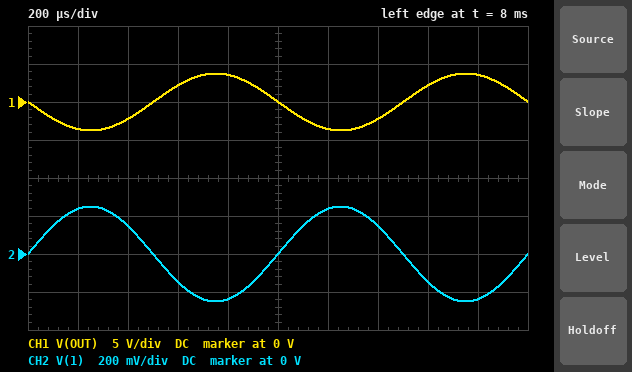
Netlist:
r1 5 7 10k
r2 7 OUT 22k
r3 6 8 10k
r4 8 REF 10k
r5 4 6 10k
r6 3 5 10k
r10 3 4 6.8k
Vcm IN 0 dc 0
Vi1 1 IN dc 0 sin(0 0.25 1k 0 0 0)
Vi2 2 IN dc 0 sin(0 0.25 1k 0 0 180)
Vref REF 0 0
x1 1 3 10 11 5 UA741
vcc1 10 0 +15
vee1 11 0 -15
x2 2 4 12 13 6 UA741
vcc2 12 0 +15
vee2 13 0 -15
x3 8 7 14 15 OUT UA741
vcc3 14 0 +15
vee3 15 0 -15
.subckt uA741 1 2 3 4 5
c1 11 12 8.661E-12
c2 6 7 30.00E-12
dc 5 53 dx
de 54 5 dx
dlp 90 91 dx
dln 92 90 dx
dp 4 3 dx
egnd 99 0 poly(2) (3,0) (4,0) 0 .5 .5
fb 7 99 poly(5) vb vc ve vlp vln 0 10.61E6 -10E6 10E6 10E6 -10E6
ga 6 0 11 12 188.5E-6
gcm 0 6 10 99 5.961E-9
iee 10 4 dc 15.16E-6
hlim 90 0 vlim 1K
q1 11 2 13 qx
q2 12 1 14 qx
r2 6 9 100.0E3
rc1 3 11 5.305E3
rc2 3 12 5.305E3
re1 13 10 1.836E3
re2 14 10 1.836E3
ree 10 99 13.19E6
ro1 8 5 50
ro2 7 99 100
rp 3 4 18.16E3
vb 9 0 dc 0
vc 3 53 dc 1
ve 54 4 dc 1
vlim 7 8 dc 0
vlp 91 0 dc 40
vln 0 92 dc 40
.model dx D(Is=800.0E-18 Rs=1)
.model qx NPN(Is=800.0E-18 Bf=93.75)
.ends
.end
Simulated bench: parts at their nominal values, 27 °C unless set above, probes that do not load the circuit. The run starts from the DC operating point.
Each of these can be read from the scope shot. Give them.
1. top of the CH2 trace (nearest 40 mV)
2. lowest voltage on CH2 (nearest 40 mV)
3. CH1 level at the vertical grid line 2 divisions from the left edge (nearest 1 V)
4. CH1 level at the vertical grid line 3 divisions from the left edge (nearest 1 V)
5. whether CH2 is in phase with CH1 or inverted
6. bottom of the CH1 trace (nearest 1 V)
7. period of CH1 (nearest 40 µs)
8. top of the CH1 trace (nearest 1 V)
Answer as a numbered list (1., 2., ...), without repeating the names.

1. 240 mV
2. -240 mV
3. -2 V
4. 2 V
5. inverted
6. -4 V
7. 1.00 ms
8. 4 V
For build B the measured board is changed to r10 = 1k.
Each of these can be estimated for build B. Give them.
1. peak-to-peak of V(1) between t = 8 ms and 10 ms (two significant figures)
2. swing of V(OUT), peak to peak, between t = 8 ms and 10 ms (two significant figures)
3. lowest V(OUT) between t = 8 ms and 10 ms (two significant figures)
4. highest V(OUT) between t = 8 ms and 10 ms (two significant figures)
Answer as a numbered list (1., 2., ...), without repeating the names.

1. 500 mV
2. 29 V
3. -15 V
4. 15 V
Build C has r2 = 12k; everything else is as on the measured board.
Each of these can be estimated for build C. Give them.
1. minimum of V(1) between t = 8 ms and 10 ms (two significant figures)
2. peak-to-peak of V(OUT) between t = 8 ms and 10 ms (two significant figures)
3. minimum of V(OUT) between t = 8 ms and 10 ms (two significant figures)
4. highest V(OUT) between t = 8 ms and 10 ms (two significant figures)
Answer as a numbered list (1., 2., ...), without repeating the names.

1. -250 mV
2. 4.5 V
3. -2.3 V
4. 2.3 V
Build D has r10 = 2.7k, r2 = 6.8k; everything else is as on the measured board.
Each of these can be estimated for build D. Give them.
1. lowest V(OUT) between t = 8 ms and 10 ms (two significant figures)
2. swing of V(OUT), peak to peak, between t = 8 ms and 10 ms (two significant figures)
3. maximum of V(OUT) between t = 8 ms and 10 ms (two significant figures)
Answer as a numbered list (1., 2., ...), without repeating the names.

1. -3.2 V
2. 6.4 V
3. 3.2 V
